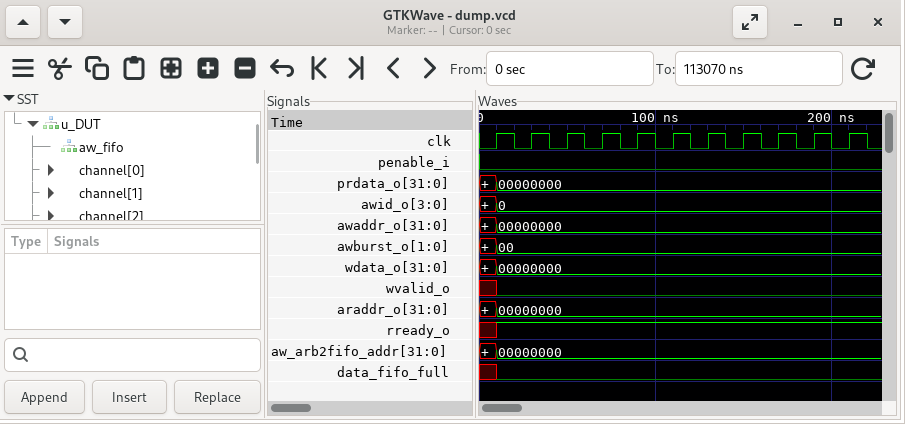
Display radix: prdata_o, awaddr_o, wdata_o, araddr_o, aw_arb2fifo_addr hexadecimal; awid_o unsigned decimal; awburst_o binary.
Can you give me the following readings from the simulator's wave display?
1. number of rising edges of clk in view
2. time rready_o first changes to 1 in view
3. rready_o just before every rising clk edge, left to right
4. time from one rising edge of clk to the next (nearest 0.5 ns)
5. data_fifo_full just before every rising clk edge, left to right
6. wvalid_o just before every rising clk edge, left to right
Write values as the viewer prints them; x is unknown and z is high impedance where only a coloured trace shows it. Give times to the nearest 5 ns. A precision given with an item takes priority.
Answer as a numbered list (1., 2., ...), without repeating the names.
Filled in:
1. 11
2. 10 ns
3. x 1 1 1 1 1 1 1 1 1 1
4. 20 ns
5. x 0 0 0 0 0 0 0 0 0 0
6. x 0 0 0 0 0 0 0 0 0 0
